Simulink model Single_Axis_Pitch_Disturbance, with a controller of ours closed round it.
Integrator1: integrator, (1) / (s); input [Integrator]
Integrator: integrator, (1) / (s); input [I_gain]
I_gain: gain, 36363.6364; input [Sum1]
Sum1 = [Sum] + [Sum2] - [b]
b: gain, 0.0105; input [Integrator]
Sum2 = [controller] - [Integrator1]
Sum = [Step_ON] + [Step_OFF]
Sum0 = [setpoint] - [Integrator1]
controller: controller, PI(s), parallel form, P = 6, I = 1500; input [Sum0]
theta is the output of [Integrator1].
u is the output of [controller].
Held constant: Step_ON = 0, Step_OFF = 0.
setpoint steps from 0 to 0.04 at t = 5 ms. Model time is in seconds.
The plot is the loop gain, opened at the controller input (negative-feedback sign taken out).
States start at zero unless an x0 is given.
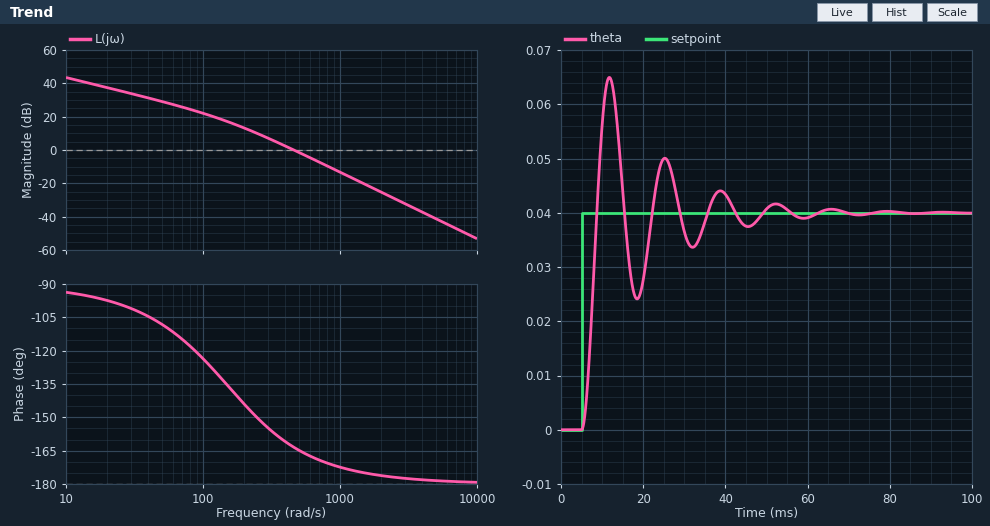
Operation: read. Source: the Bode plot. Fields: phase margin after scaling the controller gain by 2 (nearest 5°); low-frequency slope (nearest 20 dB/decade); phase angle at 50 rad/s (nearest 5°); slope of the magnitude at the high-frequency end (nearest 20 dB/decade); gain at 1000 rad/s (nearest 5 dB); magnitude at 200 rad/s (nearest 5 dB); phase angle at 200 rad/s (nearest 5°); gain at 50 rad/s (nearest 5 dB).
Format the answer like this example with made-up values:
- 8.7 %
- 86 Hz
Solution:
- 10°
- -20 dB/decade
- -110°
- -40 dB/decade
- -15 dB
- 15 dB
- -145°
- 30 dB
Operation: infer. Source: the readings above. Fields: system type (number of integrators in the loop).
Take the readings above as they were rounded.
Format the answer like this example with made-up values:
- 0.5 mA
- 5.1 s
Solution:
- 1
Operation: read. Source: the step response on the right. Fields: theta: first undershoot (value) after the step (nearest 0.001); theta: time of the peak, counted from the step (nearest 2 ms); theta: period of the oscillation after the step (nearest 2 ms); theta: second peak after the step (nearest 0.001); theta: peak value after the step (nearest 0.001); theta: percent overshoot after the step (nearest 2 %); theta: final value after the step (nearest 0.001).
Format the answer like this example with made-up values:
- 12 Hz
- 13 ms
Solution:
- 0.024
- 6 ms
- 14 ms
- 0.050
- 0.065
- 62 %
- 0.040
